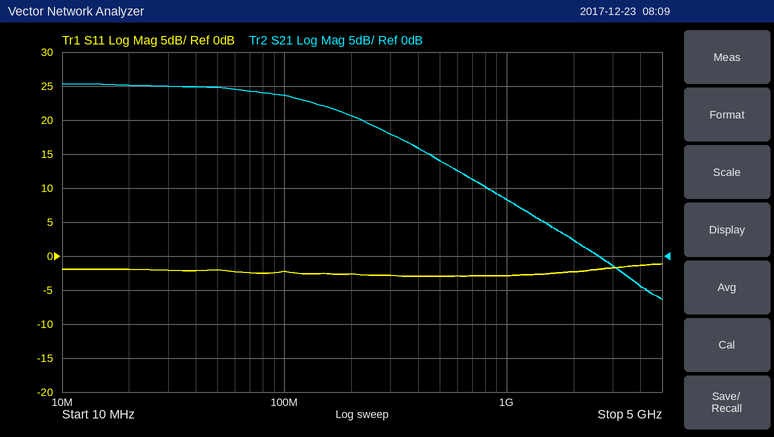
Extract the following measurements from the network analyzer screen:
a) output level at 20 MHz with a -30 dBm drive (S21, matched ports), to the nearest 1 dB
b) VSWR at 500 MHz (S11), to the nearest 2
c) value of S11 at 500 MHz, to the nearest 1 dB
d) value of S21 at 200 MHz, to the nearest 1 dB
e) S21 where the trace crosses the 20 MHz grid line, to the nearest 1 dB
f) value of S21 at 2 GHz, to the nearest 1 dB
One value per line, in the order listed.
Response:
-5 dBm
6
-3 dB
21 dB
25 dB
2 dB
